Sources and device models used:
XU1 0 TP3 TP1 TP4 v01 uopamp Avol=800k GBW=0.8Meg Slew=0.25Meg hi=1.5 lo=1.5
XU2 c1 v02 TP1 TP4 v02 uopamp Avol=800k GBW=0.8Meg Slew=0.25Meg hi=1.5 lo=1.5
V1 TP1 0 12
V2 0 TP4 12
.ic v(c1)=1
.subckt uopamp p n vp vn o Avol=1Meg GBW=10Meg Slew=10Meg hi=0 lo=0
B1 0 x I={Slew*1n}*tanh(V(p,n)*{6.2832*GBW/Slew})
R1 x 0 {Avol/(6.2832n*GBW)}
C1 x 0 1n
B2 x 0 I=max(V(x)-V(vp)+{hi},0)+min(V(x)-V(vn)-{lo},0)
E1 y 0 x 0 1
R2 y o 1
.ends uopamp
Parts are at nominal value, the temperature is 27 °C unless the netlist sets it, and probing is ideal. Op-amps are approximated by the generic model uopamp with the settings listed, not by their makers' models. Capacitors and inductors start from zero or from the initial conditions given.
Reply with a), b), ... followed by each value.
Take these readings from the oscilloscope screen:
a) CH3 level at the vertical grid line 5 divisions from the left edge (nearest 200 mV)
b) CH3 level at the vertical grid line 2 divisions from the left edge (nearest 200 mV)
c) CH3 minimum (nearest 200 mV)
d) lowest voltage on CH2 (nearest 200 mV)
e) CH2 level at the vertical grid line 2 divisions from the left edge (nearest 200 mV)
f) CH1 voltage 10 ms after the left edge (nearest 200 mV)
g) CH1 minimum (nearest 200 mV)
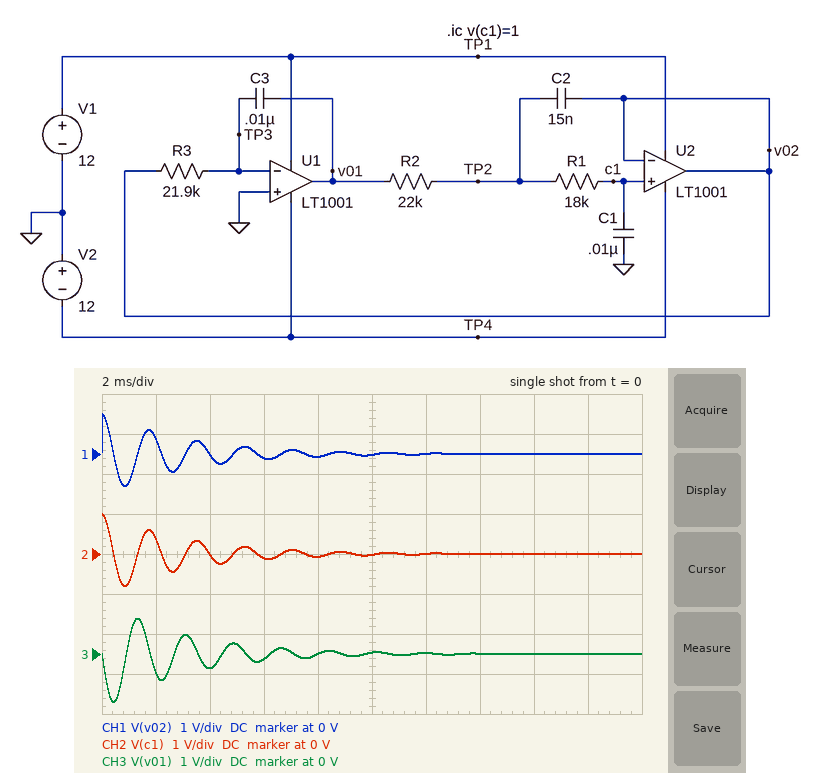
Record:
a) 0 V
b) -400 mV
c) -1.2 V
d) -800 mV
e) 0 V
f) 0 V
g) -800 mV
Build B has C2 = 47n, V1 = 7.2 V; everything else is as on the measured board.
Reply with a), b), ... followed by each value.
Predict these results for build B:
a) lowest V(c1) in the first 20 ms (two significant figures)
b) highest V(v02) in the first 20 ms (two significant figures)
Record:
a) -9.3 V
b) 5.7 V
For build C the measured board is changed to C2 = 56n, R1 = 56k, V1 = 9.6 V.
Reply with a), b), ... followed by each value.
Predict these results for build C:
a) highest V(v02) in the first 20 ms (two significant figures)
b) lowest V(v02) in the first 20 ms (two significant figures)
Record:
a) 7.2 V
b) -8.4 V
